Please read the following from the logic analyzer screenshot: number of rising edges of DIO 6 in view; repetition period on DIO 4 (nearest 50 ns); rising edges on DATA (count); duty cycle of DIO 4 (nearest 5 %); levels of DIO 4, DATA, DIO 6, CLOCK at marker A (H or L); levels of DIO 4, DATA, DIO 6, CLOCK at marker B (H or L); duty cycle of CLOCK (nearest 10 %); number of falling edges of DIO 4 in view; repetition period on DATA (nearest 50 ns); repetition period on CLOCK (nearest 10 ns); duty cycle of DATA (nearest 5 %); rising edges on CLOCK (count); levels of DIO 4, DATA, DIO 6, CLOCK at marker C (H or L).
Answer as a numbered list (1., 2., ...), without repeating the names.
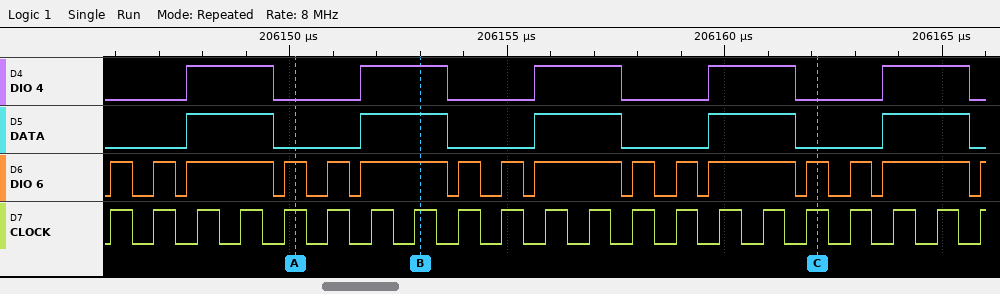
1. 16
2. 4000 ns
3. 5
4. 50 %
5. DIO 4=L, DATA=L, DIO 6=H, CLOCK=H
6. DIO 4=H, DATA=H, DIO 6=H, CLOCK=H
7. 50 %
8. 5
9. 4000 ns
10. 1000 ns
11. 50 %
12. 21
13. DIO 4=L, DATA=L, DIO 6=H, CLOCK=H
